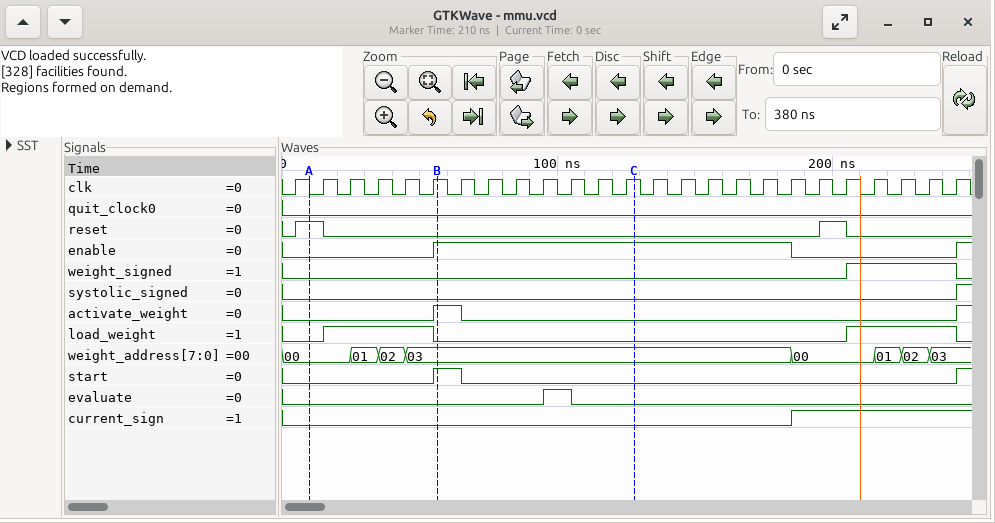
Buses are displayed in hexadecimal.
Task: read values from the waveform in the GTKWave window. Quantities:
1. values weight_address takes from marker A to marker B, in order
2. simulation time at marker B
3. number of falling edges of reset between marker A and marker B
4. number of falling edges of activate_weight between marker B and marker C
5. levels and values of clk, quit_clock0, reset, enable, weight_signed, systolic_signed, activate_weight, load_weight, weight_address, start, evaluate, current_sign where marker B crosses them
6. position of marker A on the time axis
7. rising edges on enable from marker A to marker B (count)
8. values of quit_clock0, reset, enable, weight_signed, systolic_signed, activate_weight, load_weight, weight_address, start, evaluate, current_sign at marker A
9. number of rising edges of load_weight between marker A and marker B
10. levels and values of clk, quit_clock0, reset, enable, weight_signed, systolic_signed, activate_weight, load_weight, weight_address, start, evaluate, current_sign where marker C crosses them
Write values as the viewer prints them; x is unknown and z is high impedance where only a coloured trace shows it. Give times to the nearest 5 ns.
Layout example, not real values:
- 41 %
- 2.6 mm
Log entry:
- 00, 01, 02, 03
- 55 ns
- 1
- 1
- clk=1, quit_clock0=0, reset=0, enable=1, weight_signed=0, systolic_signed=0, activate_weight=1, load_weight=0, weight_address=03, start=1, evaluate=0, current_sign=0
- 10 ns
- 1
- quit_clock0=0, reset=1, enable=0, weight_signed=0, systolic_signed=0, activate_weight=0, load_weight=0, weight_address=00, start=0, evaluate=0, current_sign=0
- 1
- clk=1, quit_clock0=0, reset=0, enable=1, weight_signed=0, systolic_signed=0, activate_weight=0, load_weight=0, weight_address=03, start=0, evaluate=0, current_sign=0
